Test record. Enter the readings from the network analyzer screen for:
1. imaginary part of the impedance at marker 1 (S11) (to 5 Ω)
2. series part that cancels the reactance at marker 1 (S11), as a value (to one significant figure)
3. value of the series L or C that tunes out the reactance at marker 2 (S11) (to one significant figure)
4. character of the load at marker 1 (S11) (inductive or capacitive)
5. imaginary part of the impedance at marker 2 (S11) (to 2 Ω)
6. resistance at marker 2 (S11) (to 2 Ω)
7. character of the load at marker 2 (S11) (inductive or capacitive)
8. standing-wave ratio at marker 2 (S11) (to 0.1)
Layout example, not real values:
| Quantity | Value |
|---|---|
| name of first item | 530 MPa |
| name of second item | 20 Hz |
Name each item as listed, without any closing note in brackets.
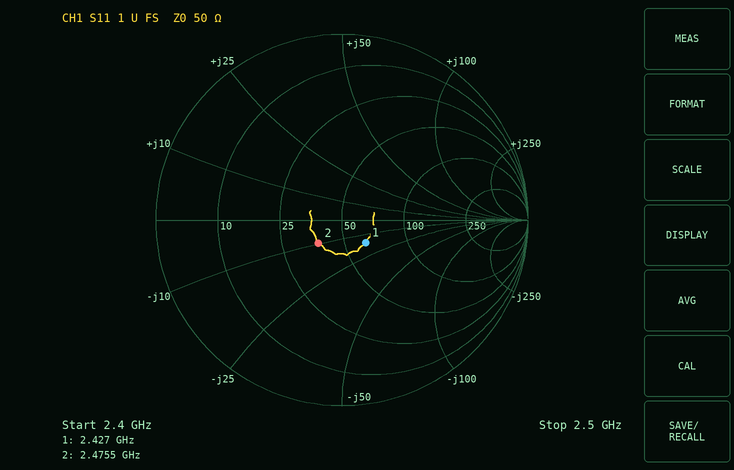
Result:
| Quantity | Value |
|---|---|
| imaginary part of the impedance at marker 1 (S11) | -15 Ω |
| series part that cancels the reactance at marker 1 (S11), as a value | 1 nH |
| value of the series L or C that tunes out the reactance at marker 2 (S11) | 600 pH |
| character of the load at marker 1 (S11) | capacitive |
| imaginary part of the impedance at marker 2 (S11) | -10 Ω |
| resistance at marker 2 (S11) | 38 Ω |
| character of the load at marker 2 (S11) | capacitive |
| standing-wave ratio at marker 2 (S11) | 1.4 |
